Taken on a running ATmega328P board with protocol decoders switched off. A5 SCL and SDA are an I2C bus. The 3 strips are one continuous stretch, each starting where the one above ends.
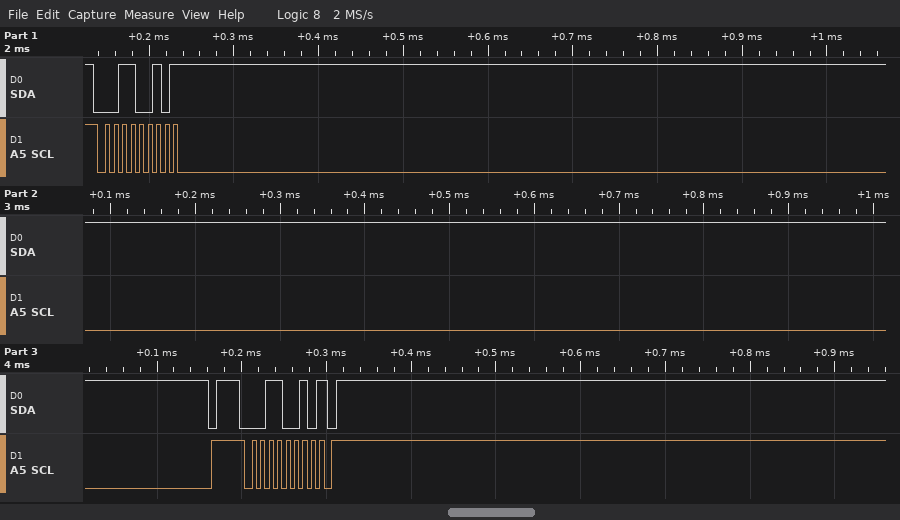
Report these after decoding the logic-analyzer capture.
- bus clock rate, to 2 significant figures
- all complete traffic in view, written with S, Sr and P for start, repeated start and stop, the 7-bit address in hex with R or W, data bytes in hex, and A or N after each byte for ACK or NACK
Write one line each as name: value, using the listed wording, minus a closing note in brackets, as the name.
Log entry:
bus clock rate, to 2 significant figures: 100 kHz
all complete traffic in view, written with S, Sr and P for start, repeated start and stop, the 7-bit address in hex with R or W, data bytes in hex, and A or N after each byte for ACK or NACK: S 19W N P S 19W N P
